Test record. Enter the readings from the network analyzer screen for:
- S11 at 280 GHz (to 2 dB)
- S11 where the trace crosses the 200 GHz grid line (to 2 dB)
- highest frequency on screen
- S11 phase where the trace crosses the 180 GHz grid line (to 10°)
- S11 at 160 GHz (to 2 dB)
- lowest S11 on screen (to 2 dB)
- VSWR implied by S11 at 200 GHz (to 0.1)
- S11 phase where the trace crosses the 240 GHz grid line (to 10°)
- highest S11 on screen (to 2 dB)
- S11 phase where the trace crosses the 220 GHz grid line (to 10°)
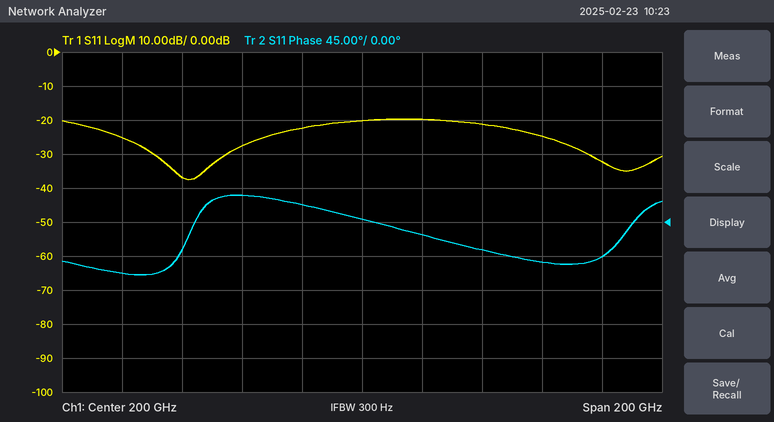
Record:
-32 dB
-20 dB
300 GHz
20°
-28 dB
-38 dB
1.2
-40°
-20 dB
-20°
